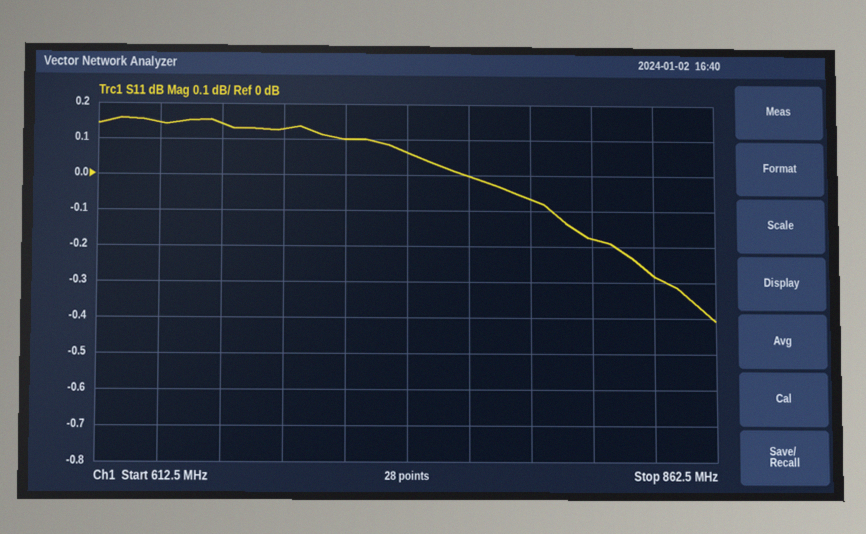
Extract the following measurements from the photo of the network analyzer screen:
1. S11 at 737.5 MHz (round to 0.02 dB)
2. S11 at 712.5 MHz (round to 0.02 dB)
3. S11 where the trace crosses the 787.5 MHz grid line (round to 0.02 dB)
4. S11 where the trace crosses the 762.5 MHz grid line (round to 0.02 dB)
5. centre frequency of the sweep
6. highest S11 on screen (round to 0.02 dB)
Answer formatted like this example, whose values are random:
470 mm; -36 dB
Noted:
0.06 dB; 0.10 dB; -0.06 dB; 0.00 dB; 737.5 MHz; 0.16 dB
